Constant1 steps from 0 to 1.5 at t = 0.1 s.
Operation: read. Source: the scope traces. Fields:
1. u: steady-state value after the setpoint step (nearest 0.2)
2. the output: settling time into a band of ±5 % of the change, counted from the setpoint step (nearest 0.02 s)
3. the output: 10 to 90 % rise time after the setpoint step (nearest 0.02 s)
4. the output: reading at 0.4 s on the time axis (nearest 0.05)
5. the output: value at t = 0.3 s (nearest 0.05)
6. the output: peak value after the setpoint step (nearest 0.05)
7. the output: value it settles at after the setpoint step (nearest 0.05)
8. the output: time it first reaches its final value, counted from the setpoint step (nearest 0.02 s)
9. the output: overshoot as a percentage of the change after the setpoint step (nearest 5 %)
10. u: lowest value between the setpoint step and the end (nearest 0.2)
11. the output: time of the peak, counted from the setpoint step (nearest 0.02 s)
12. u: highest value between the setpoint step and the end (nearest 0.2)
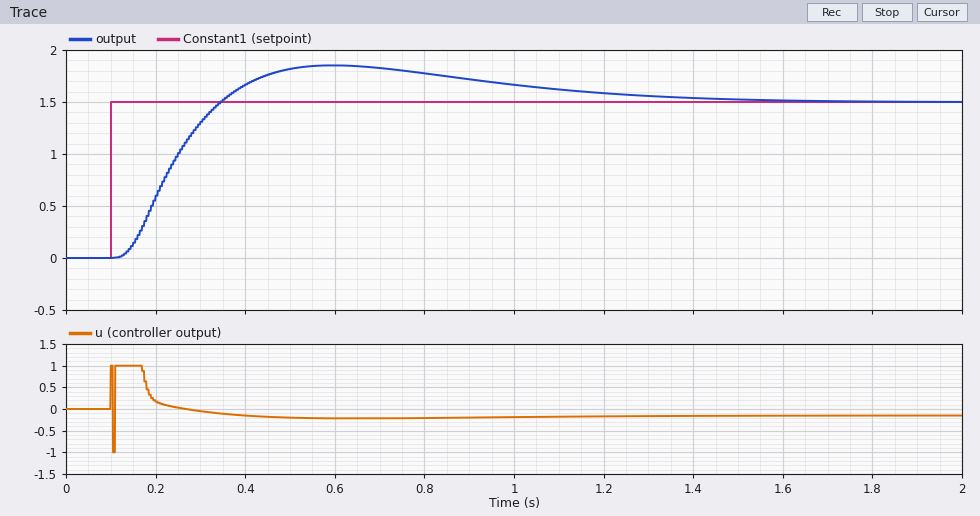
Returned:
-0.2
1.14 s
0.16 s
1.65
1.30
1.85
1.50
0.24 s
25 %
-1.0
0.50 s
1.0
